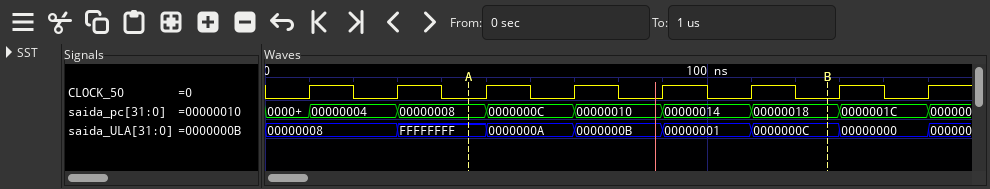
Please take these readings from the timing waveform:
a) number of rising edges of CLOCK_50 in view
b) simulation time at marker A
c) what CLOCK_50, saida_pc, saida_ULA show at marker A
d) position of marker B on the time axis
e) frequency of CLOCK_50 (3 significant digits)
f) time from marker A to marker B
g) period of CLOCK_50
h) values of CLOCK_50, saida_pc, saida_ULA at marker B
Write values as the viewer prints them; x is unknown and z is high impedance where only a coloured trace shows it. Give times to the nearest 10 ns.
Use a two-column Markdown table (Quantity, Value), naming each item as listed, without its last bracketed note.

| Quantity | Value |
|---|---|
| number of rising edges of CLOCK_50 in view | 8 |
| simulation time at marker A | 50 ns |
| what CLOCK_50, saida_pc, saida_ULA show at marker A | CLOCK_50=0, saida_pc=00000008, saida_ULA=FFFFFFFF |
| position of marker B on the time axis | 130 ns |
| frequency of CLOCK_50 | 50.0 MHz |
| time from marker A to marker B | 80 ns |
| period of CLOCK_50 | 20 ns |
| values of CLOCK_50, saida_pc, saida_ULA at marker B | CLOCK_50=0, saida_pc=00000018, saida_ULA=0000000C |
